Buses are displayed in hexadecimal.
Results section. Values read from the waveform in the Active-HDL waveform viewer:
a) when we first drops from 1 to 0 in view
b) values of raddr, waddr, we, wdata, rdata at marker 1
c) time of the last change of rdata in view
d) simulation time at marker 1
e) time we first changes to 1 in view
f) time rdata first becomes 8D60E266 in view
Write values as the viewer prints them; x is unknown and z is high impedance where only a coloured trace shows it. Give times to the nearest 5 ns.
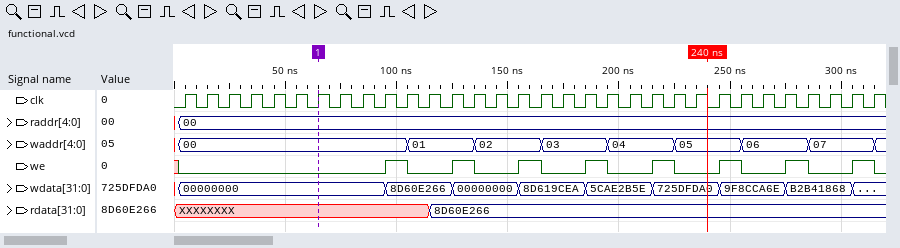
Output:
105 ns
raddr=00, waddr=00, we=0, wdata=00000000, rdata=XXXXXXXX
115 ns
65 ns
95 ns
115 ns
